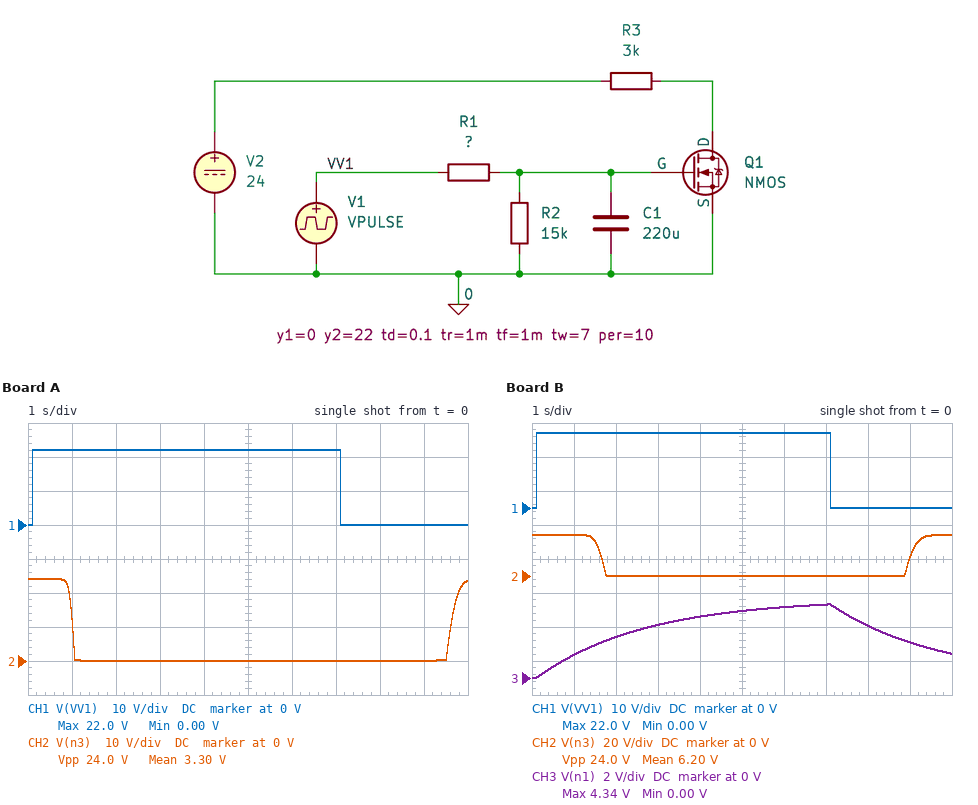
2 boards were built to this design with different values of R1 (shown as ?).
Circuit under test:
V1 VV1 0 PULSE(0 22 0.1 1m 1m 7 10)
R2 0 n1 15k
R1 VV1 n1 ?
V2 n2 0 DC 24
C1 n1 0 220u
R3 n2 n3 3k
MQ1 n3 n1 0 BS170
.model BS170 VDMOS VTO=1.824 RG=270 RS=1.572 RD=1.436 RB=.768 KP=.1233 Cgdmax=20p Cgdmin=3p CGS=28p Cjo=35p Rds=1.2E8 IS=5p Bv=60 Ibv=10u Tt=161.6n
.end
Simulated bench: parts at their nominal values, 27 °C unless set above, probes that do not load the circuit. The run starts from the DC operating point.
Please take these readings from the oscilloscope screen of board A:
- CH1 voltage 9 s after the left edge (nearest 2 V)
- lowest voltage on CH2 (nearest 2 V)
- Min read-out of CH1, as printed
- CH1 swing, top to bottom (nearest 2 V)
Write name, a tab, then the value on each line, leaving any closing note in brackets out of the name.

CH1 voltage 9 s after the left edge	0 V
lowest voltage on CH2	0 V
Min read-out of CH1, as printed	0.00 V
CH1 swing, top to bottom	22 V
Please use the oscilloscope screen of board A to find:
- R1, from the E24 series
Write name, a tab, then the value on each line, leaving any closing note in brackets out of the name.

R1, from the E24 series	36 kΩ
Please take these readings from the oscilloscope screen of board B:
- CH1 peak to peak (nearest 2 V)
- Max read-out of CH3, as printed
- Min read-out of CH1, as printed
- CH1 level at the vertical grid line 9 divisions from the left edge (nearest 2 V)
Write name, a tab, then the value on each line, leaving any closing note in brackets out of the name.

CH1 peak to peak	22 V
Max read-out of CH3, as printed	4.34 V
Min read-out of CH1, as printed	0.00 V
CH1 level at the vertical grid line 9 divisions from the left edge	0 V
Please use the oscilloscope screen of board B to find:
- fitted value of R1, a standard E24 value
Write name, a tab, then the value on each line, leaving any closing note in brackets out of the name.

fitted value of R1, a standard E24 value	56 kΩ
